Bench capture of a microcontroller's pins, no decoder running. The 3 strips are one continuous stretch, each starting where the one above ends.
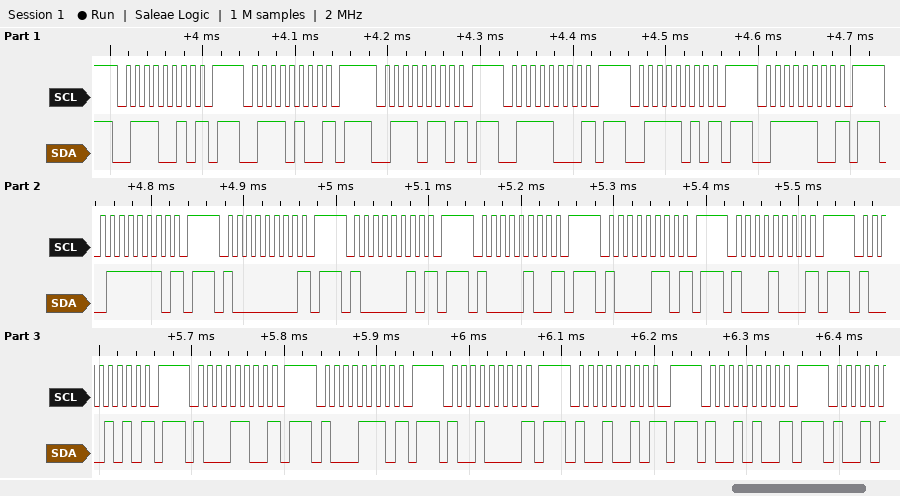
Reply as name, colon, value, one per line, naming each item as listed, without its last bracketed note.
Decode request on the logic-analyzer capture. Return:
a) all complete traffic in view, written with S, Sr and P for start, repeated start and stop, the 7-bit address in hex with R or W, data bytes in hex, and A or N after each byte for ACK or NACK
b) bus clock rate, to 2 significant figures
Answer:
all complete traffic in view, written with S, Sr and P for start, repeated start and stop, the 7-bit address in hex with R or W, data bytes in hex, and A or N after each byte for ACK or NACK: S 39W N P S 3AW N P S 3BW N P S 3CW N P S 3DW N P S 3EW N P S 3FW N P S 40W N P S 41W N P S 42W N P S 43W N P S 44W N P S 45W N P S 46W N P S 47W N P S 48W N P S 49W N P S 4AW N P
bus clock rate, to 2 significant figures: 100 kHz
